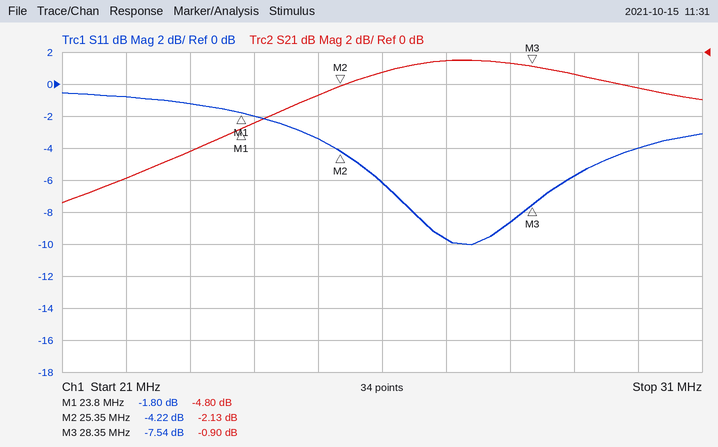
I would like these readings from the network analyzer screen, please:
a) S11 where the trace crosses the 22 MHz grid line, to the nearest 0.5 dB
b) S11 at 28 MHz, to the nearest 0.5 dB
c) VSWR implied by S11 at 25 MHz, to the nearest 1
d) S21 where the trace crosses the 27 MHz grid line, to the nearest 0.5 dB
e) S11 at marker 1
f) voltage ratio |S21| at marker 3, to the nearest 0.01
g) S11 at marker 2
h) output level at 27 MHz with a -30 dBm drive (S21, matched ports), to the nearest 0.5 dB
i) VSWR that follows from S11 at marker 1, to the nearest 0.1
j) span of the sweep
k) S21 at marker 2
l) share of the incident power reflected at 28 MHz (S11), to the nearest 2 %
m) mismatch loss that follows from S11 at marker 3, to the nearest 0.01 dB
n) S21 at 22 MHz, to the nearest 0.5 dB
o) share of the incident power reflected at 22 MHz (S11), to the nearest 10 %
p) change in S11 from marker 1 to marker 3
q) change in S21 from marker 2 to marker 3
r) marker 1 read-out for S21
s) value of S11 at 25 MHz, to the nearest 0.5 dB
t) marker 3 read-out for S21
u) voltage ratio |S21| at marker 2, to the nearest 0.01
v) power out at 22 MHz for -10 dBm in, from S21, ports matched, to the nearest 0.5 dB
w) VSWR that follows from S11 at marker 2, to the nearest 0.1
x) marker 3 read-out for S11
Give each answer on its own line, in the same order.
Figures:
-1.0 dB
-8.5 dB
5
-0.5 dB
-1.80 dB
0.90
-4.22 dB
-30.5 dBm
9.7
10 MHz
-2.13 dB
14 %
0.84 dB
-8.0 dB
80 %
-5.74 dB
1.23 dB
-4.80 dB
-3.5 dB
-0.90 dB
0.78
-18.0 dBm
4.2
-7.54 dB
